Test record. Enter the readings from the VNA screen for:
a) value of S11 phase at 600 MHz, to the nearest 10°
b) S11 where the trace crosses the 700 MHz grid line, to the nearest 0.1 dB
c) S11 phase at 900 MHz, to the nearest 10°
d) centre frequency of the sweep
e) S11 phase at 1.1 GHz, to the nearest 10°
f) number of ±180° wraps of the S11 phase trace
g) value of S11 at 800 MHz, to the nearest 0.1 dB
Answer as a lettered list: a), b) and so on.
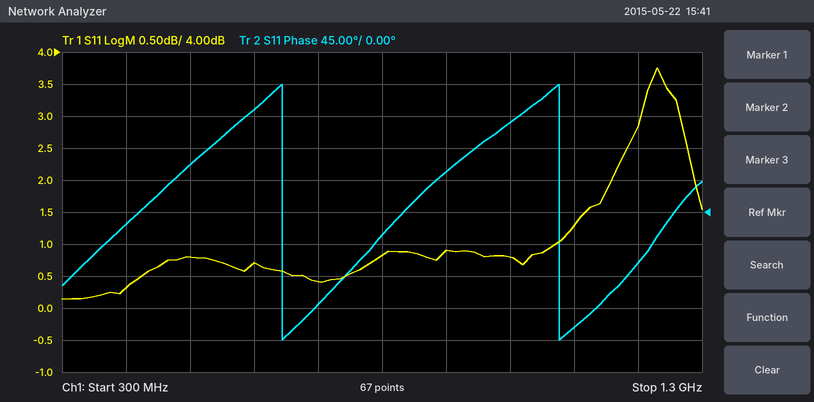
a) 140°
b) 0.4 dB
c) 60°
d) 800 MHz
e) -160°
f) 2
g) 0.8 dB
